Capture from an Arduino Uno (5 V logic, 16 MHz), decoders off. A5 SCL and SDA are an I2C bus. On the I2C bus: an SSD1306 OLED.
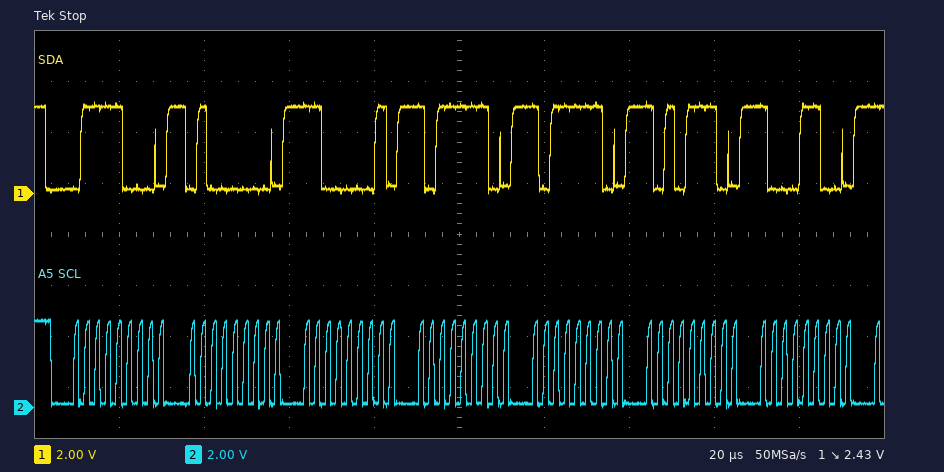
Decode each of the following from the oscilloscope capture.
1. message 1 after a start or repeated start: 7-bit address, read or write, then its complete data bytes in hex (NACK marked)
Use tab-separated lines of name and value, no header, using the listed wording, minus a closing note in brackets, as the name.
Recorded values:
message 1 after a start or repeated start: 7-bit address, read or write, then its complete data bytes in hex	0x3C write: 40 C1 BE BE AE 8C
